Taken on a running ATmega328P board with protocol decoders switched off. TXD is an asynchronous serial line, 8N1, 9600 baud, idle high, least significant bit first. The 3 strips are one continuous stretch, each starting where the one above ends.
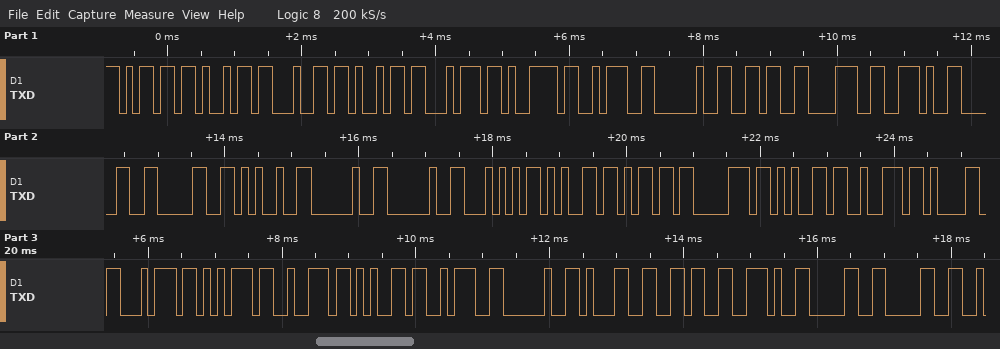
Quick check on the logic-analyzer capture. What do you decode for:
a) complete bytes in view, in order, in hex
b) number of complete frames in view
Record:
6D 69 64 69 74 79 3A 20 36 38 2E 30 30 25 20 20 54 65 6D 70 65 72 61 74 75 72 65 3A 20 31 36 2E 30 30
34
